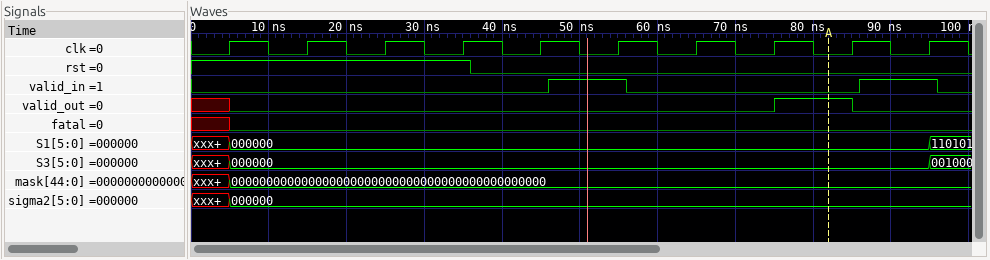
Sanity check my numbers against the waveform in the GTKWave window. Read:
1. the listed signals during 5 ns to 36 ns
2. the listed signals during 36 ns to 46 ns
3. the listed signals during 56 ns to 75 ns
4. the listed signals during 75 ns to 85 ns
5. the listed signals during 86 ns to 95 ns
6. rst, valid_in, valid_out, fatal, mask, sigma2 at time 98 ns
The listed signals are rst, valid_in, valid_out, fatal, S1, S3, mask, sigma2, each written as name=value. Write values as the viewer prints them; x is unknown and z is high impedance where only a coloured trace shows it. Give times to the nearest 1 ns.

rst=1, valid_in=0, valid_out=0, fatal=0, S1=000000, S3=000000, mask=000000000000000000000000000000000000000000000, sigma2=000000
rst=0, valid_in=0, valid_out=0, fatal=0, S1=000000, S3=000000, mask=000000000000000000000000000000000000000000000, sigma2=000000
rst=0, valid_in=0, valid_out=0, fatal=0, S1=000000, S3=000000, mask=000000000000000000000000000000000000000000000, sigma2=000000
rst=0, valid_in=0, valid_out=1, fatal=0, S1=000000, S3=000000, mask=000000000000000000000000000000000000000000000, sigma2=000000
rst=0, valid_in=1, valid_out=0, fatal=0, S1=000000, S3=000000, mask=000000000000000000000000000000000000000000000, sigma2=000000
rst=0, valid_in=0, valid_out=0, fatal=0, mask=000000000000000000000000000000000000000000000, sigma2=000000
